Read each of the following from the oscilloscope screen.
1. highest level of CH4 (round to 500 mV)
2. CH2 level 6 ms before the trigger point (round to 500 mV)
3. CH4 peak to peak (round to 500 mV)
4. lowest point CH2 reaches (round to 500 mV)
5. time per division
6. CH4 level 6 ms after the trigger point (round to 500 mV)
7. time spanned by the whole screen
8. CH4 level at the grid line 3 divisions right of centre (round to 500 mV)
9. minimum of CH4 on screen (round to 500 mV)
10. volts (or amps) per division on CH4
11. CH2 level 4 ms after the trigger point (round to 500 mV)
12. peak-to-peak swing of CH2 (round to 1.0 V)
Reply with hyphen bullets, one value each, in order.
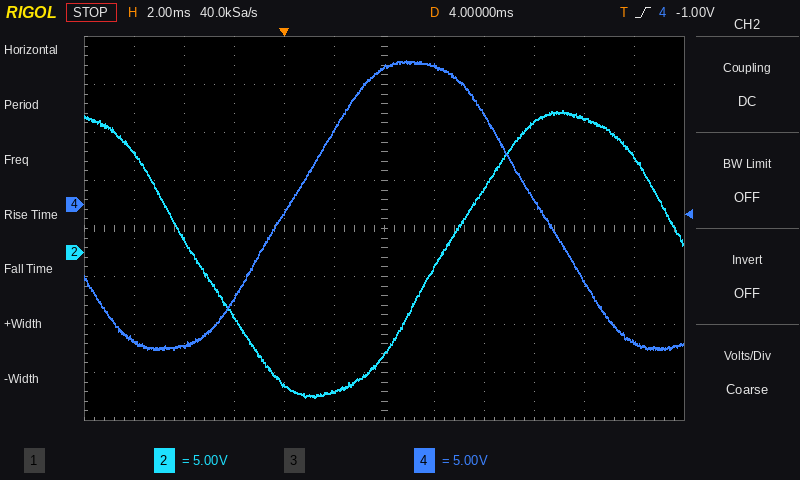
- 15.0 V
- 10.5 V
- 30.0 V
- -15.0 V
- 2 ms
- 14.5 V
- 24 ms
- 500 mV
- -15.0 V
- 5 V
- -10.5 V
- 30.0 V
